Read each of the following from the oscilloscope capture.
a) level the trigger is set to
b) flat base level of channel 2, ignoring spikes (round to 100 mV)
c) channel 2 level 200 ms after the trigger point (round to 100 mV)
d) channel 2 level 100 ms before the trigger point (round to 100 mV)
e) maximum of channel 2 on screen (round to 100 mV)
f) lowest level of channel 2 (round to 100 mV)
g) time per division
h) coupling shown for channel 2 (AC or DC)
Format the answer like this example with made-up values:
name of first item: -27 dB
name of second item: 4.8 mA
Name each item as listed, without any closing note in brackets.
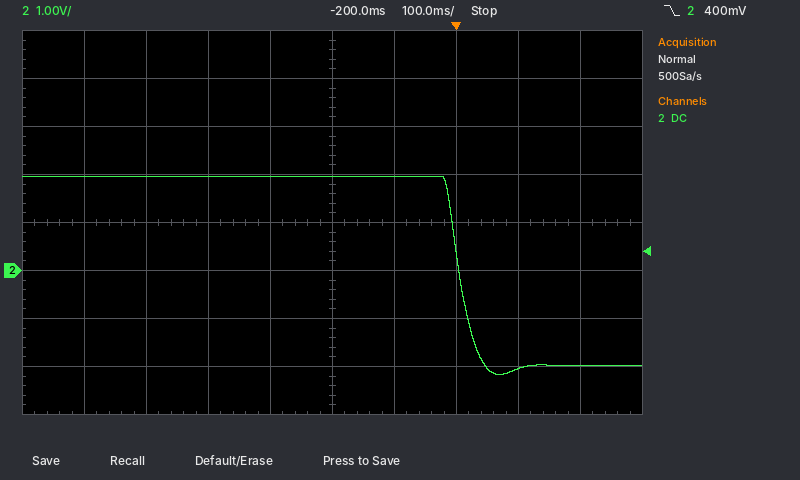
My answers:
level the trigger is set to: 400 mV
flat base level of channel 2, ignoring spikes: -2.0 V
channel 2 level 200 ms after the trigger point: -2.0 V
channel 2 level 100 ms before the trigger point: 2.0 V
maximum of channel 2 on screen: 2.0 V
lowest level of channel 2: -2.2 V
time per division: 100 ms
coupling shown for channel 2: DC
